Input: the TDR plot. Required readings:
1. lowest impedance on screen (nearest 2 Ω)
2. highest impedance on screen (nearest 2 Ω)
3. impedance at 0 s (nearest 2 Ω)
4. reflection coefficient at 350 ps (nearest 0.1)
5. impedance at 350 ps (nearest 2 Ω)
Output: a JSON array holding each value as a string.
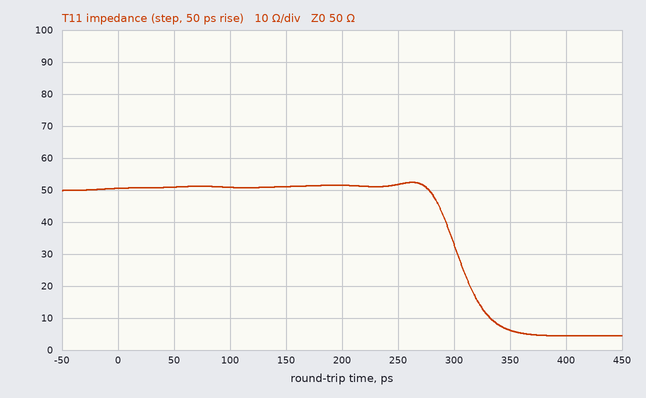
["4 Ω", "52 Ω", "50 Ω", "-0.8", "6 Ω"]
